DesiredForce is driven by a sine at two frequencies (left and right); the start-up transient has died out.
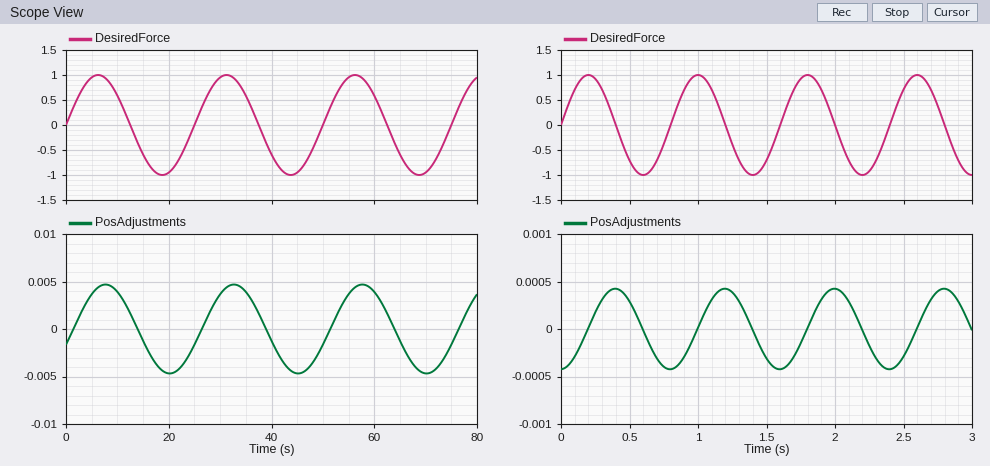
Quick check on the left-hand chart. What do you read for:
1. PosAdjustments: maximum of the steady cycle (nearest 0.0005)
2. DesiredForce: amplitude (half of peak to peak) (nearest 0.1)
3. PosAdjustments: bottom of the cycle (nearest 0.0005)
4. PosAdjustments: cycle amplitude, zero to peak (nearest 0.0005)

0.0045
1.0
-0.0045
0.0045
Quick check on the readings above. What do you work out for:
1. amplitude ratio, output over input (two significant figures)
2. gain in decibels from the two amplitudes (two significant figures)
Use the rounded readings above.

0.0045
-47 dB
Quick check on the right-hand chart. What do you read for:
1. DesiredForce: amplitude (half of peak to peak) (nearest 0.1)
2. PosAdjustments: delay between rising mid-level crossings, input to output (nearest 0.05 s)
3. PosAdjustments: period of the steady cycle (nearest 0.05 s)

1.0
0.20 s
0.80 s
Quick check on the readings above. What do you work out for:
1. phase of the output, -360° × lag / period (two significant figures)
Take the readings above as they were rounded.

-90°
